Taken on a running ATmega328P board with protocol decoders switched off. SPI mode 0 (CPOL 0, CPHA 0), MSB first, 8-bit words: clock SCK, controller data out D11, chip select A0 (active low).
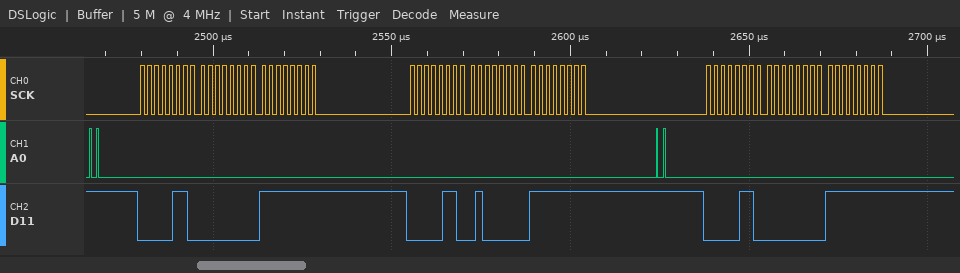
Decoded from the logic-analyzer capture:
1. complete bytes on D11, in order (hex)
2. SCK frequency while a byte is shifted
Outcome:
06 00 FF 06 40 FF 06 00 FF
500 kHz
